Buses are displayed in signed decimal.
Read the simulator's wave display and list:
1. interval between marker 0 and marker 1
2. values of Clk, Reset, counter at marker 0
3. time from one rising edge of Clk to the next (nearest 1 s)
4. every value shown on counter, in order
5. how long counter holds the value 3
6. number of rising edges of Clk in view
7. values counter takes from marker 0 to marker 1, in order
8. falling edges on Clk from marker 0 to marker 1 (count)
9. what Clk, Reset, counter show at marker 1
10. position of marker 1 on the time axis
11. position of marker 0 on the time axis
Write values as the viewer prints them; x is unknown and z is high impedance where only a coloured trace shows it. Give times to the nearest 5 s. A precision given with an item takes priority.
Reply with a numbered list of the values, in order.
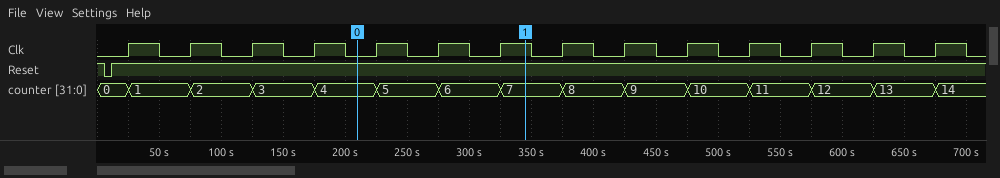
1. 135 s
2. Clk=0, Reset=1, counter=4
3. 50 s
4. 0, 1, 2, 3, 4, 5, 6, 7, 8, 9, 10, 11, 12, 13, 14
5. 50 s
6. 14
7. 4, 5, 6, 7
8. 2
9. Clk=1, Reset=1, counter=7
10. 345 s
11. 210 s
